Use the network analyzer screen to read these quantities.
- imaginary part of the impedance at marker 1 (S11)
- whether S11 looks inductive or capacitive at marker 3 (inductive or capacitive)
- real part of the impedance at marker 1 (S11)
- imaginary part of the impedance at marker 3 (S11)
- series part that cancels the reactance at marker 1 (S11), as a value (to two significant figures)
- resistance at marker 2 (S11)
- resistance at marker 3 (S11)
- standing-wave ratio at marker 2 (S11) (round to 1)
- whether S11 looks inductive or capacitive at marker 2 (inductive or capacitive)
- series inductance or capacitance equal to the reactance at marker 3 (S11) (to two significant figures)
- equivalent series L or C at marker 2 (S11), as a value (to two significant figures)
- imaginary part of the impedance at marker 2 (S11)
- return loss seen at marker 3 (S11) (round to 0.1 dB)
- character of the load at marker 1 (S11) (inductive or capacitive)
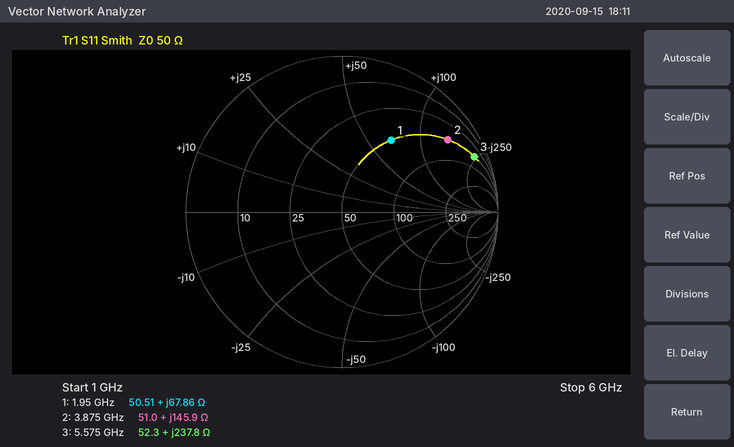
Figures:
+67.86 Ω
inductive
50.51 Ω
+237.8 Ω
1.2 pF
51.0 Ω
52.3 Ω
10
inductive
6.8 nH
6.0 nH
+145.9 Ω
0.7 dB
inductive
